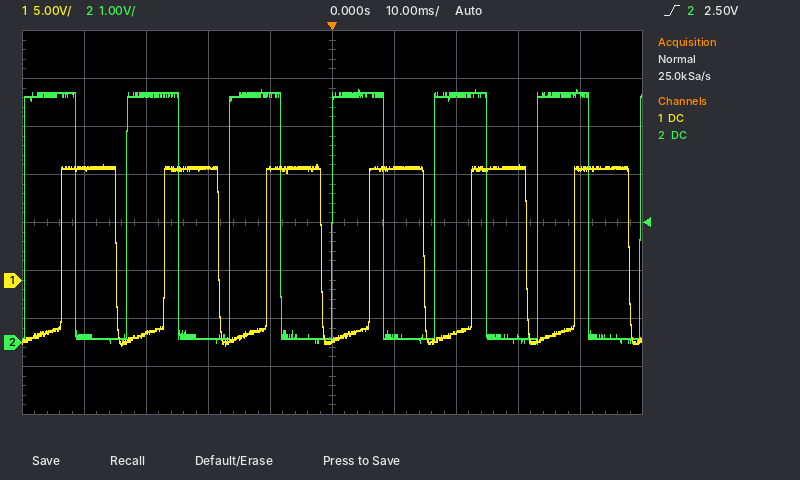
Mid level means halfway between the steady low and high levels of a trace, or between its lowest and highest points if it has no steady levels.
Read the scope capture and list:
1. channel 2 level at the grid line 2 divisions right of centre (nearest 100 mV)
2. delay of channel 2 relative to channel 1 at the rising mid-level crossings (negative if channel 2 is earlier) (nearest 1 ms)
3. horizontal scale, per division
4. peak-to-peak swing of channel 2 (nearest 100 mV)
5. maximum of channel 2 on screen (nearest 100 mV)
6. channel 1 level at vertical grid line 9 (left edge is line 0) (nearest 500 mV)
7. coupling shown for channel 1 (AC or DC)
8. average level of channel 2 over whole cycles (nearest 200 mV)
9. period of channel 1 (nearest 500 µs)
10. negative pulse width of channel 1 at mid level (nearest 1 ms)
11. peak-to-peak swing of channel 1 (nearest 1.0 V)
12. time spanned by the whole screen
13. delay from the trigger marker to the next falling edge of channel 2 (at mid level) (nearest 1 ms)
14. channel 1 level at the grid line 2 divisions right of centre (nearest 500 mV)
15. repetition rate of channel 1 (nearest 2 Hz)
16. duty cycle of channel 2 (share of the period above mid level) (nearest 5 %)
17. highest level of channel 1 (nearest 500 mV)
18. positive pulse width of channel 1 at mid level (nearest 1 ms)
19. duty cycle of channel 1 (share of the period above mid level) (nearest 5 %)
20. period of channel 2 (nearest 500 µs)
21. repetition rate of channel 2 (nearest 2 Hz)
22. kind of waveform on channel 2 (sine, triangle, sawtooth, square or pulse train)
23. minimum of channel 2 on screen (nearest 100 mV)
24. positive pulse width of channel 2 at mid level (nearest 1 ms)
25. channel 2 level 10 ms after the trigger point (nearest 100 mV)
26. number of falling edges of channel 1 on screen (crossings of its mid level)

5.2 V
-6 ms
10 ms
5.3 V
5.3 V
11.5 V
DC
2.6 V
16.5 ms
8 ms
19.0 V
100 ms
8 ms
-5.5 V
60 Hz
50 %
12.0 V
9 ms
55 %
16.5 ms
60 Hz
square
0.0 V
8 ms
100 mV
6
